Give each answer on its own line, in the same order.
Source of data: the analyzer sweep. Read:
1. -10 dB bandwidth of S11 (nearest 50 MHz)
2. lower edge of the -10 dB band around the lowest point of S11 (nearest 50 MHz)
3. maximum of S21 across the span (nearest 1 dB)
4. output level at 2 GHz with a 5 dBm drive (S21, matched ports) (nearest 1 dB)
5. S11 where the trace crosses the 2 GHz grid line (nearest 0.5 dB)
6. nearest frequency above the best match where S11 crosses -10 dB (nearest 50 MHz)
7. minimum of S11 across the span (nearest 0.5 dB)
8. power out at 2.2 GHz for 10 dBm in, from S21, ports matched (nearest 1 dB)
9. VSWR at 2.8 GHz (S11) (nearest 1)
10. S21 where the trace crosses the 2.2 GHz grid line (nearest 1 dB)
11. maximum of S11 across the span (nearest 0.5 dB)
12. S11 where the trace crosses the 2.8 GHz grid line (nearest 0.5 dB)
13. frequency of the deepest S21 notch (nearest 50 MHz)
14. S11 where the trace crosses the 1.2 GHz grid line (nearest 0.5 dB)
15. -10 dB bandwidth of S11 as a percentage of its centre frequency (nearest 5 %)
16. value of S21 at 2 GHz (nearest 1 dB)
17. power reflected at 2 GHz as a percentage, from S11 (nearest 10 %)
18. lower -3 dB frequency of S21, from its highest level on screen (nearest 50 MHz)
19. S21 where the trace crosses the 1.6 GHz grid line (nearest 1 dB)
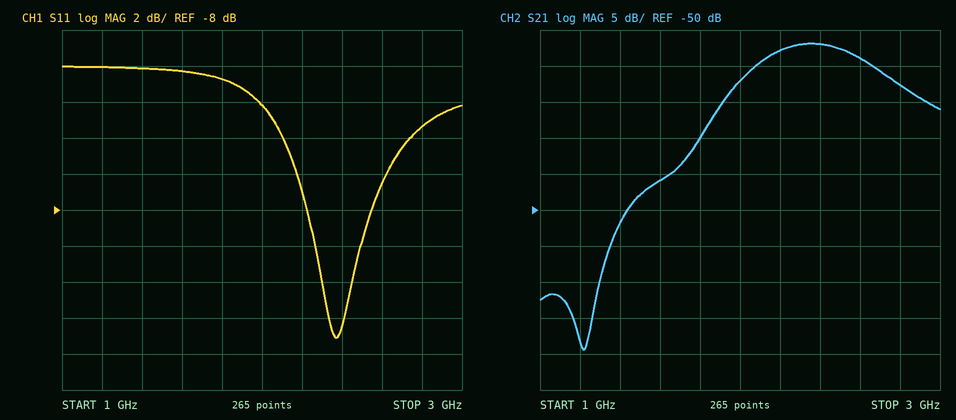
250 MHz
2.25 GHz
-27 dB
-27 dBm
-2.0 dB
2.50 GHz
-15.0 dB
-18 dBm
5
-28 dB
0.0 dB
-3.5 dB
1.20 GHz
0.0 dB
10 %
-32 dB
60 %
2.10 GHz
-46 dB
